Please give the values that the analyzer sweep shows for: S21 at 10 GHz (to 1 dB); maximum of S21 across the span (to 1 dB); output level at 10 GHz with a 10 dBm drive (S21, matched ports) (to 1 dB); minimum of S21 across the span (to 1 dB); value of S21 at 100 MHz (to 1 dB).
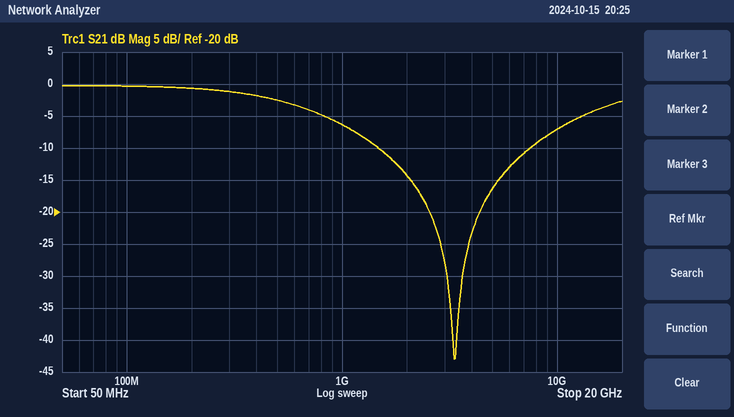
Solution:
-7 dB
0 dB
3 dBm
-43 dB
0 dB
